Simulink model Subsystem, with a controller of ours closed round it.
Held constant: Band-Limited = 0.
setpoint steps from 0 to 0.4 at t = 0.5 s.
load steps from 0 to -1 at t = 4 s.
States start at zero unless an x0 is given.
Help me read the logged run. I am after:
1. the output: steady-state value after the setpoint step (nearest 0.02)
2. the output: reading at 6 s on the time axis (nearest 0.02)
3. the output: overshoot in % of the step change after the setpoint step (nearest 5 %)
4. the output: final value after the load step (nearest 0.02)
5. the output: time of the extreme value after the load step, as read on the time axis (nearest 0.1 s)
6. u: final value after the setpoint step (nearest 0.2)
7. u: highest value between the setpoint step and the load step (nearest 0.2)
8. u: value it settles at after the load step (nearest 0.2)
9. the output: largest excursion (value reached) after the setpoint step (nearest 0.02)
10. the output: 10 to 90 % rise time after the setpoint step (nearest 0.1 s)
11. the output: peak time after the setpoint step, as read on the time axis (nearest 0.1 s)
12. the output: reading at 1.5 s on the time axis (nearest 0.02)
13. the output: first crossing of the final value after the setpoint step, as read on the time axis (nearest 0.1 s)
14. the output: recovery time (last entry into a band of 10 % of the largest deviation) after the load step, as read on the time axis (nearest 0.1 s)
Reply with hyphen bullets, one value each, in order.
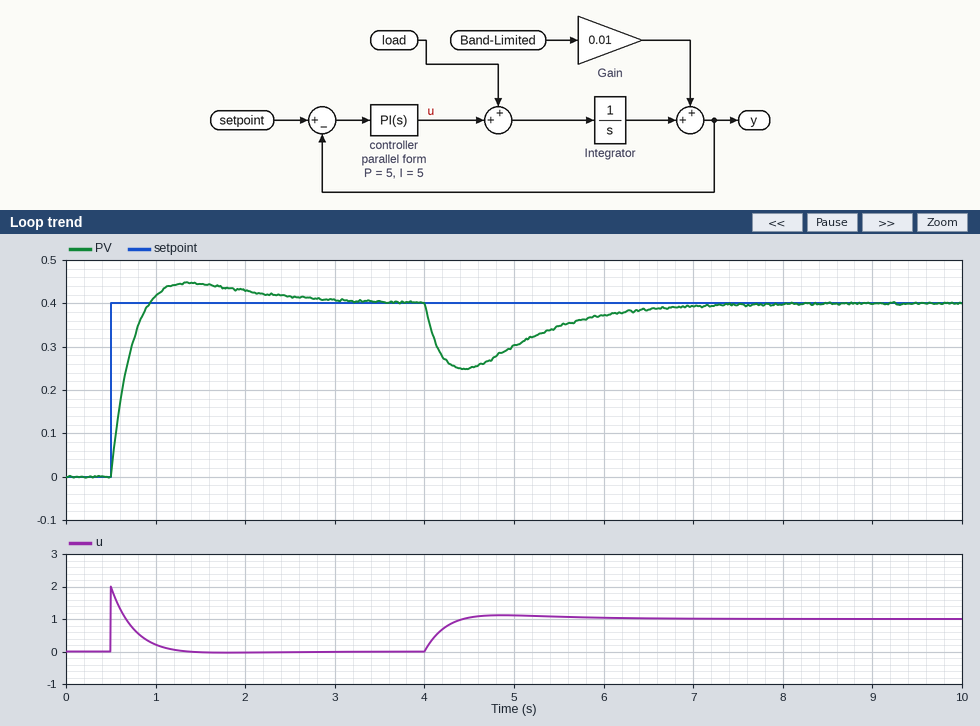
- 0.40
- 0.38
- 10 %
- 0.40
- 4.4 s
- 0.0
- 2.0
- 1.0
- 0.44
- 0.3 s
- 1.4 s
- 0.44
- 0.9 s
- 6.4 s
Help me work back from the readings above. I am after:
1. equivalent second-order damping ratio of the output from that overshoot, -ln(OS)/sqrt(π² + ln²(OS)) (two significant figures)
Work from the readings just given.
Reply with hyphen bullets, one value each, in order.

- 0.59
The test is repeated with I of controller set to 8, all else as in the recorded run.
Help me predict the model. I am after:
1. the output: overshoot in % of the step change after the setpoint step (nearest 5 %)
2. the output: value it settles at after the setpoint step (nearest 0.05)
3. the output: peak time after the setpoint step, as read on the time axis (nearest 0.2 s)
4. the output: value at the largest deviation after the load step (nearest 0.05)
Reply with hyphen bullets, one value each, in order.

- 15 %
- 0.40
- 1.2 s
- 0.25
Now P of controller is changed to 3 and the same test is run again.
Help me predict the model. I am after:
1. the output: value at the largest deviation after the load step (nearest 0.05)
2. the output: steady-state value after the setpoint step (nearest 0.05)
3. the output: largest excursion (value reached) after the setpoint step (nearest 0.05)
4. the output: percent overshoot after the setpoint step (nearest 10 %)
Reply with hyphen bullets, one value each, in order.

- 0.20
- 0.40
- 0.50
- 20 %
